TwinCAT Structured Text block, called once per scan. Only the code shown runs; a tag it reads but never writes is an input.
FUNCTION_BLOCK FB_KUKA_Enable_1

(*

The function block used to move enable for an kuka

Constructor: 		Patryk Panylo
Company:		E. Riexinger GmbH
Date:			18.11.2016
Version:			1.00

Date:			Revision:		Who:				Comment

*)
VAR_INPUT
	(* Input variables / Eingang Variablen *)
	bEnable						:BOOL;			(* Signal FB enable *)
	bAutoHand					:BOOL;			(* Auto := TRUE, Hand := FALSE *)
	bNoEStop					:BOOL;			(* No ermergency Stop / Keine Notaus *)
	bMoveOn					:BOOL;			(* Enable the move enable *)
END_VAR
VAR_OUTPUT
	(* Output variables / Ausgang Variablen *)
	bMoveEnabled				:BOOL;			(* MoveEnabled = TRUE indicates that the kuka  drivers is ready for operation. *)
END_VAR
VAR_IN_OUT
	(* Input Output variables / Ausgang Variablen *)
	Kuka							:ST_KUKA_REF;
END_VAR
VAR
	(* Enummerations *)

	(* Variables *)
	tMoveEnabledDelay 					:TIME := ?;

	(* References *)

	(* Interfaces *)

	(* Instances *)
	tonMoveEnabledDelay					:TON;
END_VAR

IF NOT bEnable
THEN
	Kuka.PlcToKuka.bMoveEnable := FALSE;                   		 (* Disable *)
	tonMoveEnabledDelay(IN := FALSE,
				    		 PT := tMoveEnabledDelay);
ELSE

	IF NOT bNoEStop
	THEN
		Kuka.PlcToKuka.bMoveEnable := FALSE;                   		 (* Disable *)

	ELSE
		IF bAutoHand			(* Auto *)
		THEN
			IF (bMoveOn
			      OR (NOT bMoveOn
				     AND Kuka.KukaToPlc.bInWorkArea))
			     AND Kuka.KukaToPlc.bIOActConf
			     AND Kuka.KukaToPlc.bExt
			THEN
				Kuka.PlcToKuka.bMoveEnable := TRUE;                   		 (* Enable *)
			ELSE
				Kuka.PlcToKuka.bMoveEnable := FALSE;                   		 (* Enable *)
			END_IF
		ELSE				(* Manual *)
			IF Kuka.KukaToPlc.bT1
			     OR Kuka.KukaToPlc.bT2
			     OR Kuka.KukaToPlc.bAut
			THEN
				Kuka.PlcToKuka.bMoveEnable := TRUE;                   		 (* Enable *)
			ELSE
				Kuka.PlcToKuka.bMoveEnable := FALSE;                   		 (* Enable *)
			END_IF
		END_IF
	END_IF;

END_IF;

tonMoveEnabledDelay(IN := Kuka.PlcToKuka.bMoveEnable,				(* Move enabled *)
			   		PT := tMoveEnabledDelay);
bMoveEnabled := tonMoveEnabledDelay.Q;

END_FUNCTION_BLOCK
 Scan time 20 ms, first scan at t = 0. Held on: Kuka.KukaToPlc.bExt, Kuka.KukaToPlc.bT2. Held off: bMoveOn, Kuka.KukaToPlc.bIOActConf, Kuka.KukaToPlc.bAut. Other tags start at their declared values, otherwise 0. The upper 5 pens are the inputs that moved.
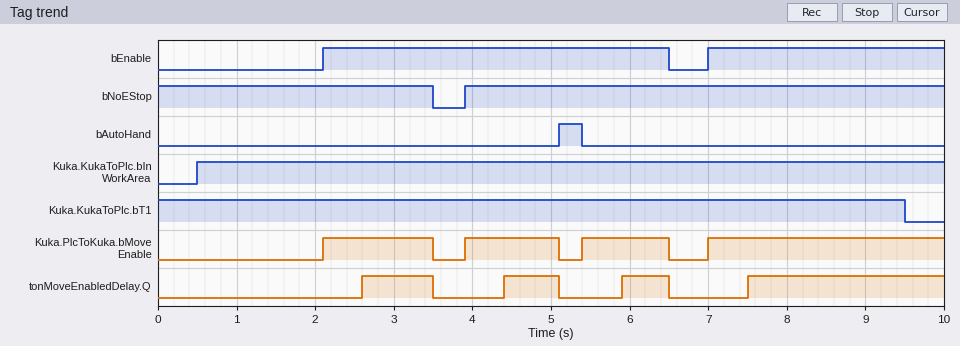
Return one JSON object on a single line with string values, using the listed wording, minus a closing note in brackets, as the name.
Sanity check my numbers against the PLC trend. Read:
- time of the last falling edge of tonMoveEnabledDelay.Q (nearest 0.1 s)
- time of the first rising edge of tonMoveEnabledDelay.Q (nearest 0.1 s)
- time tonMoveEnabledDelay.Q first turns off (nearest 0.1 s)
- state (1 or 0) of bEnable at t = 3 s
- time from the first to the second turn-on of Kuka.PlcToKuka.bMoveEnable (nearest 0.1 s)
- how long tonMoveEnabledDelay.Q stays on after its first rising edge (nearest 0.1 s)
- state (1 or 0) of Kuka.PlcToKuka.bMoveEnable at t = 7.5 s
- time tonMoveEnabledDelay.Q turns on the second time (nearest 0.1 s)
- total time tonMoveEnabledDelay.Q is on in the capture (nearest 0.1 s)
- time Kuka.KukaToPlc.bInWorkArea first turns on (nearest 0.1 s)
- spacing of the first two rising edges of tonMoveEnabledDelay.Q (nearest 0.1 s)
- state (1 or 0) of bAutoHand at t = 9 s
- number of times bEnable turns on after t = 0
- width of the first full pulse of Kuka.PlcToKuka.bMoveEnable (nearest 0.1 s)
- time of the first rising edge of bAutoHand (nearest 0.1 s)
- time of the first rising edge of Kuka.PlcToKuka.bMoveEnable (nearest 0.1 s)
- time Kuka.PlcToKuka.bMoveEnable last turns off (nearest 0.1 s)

{"time of the last falling edge of tonMoveEnabledDelay.Q": "6.5 s", "time of the first rising edge of tonMoveEnabledDelay.Q": "2.6 s", "time tonMoveEnabledDelay.Q first turns off": "3.5 s", "state (1 or 0) of bEnable at t = 3 s": "1", "time from the first to the second turn-on of Kuka.PlcToKuka.bMoveEnable": "1.8 s", "how long tonMoveEnabledDelay.Q stays on after its first rising edge": "0.9 s", "state (1 or 0) of Kuka.PlcToKuka.bMoveEnable at t = 7.5 s": "1", "time tonMoveEnabledDelay.Q turns on the second time": "4.4 s", "total time tonMoveEnabledDelay.Q is on in the capture": "4.7 s", "time Kuka.KukaToPlc.bInWorkArea first turns on": "0.5 s", "spacing of the first two rising edges of tonMoveEnabledDelay.Q": "1.8 s", "state (1 or 0) of bAutoHand at t = 9 s": "0", "number of times bEnable turns on after t = 0": "2", "width of the first full pulse of Kuka.PlcToKuka.bMoveEnable": "1.4 s", "time of the first rising edge of bAutoHand": "5.1 s", "time of the first rising edge of Kuka.PlcToKuka.bMoveEnable": "2.1 s", "time Kuka.PlcToKuka.bMoveEnable last turns off": "6.5 s"}
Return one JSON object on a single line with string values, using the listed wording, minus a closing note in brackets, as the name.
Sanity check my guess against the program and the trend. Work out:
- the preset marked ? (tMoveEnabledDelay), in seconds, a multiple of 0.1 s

{"the preset marked ? (tMoveEnabledDelay), in seconds, a multiple of 0.1 s": "0.5 s"}
